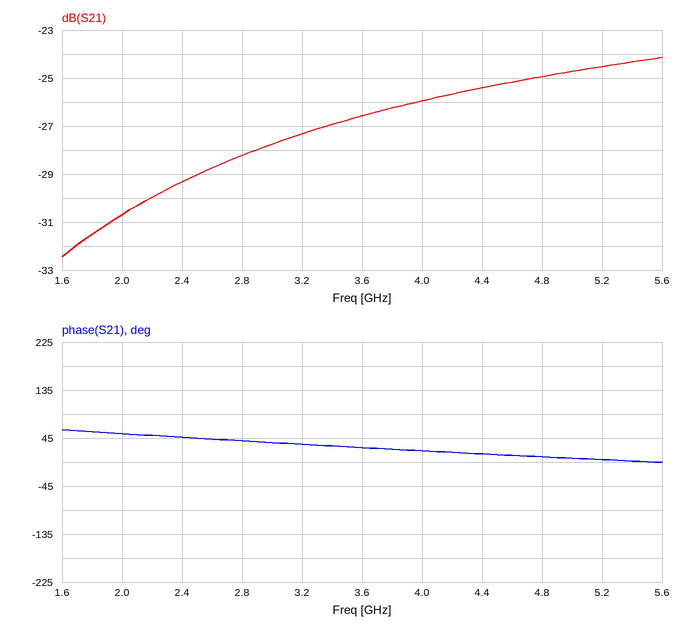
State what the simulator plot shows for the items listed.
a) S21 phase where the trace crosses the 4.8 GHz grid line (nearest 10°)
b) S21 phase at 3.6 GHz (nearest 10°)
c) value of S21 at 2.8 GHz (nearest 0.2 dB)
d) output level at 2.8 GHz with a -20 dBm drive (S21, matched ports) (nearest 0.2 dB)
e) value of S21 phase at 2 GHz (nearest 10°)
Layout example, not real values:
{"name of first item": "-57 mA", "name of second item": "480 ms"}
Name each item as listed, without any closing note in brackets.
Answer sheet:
{"S21 phase where the trace crosses the 4.8 GHz grid line": "10°", "S21 phase at 3.6 GHz": "30°", "value of S21 at 2.8 GHz": "-28.2 dB", "output level at 2.8 GHz with a -20 dBm drive (S21, matched ports)": "-48.2 dBm", "value of S21 phase at 2 GHz": "50°"}
